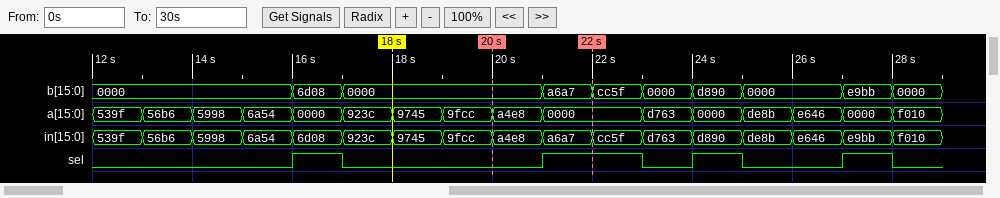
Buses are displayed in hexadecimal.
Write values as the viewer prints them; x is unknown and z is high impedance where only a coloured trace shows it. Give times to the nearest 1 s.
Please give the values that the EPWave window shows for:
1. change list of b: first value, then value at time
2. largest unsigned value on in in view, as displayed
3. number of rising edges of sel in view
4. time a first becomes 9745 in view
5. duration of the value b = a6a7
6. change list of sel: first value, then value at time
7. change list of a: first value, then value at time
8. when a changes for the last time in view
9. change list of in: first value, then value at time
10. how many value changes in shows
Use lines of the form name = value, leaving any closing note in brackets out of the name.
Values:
change list of b: first value, then value at time = 0000, 6d08 at 16 s, 0000 at 17 s, a6a7 at 21 s, cc5f at 22 s, 0000 at 23 s, d890 at 24 s, 0000 at 25 s, e9bb at 27 s, 0000 at 28 s
largest unsigned value on in in view, as displayed = f010
number of rising edges of sel in view = 4
time a first becomes 9745 in view = 18 s
duration of the value b = a6a7 = 1 s
change list of sel: first value, then value at time = 0, 1 at 16 s, 0 at 17 s, 1 at 21 s, 0 at 23 s, 1 at 24 s, 0 at 25 s, 1 at 27 s, 0 at 28 s
change list of a: first value, then value at time = 539f, 56b6 at 13 s, 5998 at 14 s, 6a54 at 15 s, 0000 at 16 s, 923c at 17 s, 9745 at 18 s, 9fcc at 19 s, a4e8 at 20 s, 0000 at 21 s, d763 at 23 s, 0000 at 24 s, de8b at 25 s, e646 at 26 s, 0000 at 27 s, f010 at 28 s
when a changes for the last time in view = 28 s
change list of in: first value, then value at time = 539f, 56b6 at 13 s, 5998 at 14 s, 6a54 at 15 s, 6d08 at 16 s, 923c at 17 s, 9745 at 18 s, 9fcc at 19 s, a4e8 at 20 s, a6a7 at 21 s, cc5f at 22 s, d763 at 23 s, d890 at 24 s, de8b at 25 s, e646 at 26 s, e9bb at 27 s, f010 at 28 s
how many value changes in shows = 16
